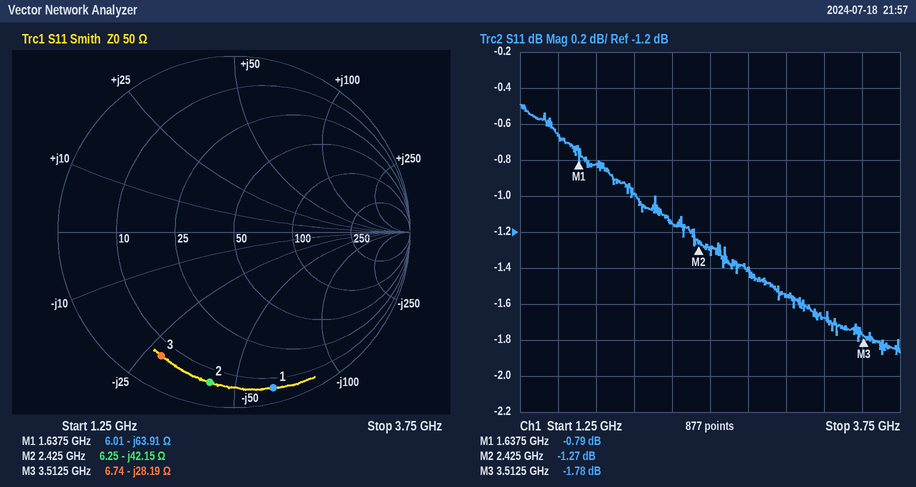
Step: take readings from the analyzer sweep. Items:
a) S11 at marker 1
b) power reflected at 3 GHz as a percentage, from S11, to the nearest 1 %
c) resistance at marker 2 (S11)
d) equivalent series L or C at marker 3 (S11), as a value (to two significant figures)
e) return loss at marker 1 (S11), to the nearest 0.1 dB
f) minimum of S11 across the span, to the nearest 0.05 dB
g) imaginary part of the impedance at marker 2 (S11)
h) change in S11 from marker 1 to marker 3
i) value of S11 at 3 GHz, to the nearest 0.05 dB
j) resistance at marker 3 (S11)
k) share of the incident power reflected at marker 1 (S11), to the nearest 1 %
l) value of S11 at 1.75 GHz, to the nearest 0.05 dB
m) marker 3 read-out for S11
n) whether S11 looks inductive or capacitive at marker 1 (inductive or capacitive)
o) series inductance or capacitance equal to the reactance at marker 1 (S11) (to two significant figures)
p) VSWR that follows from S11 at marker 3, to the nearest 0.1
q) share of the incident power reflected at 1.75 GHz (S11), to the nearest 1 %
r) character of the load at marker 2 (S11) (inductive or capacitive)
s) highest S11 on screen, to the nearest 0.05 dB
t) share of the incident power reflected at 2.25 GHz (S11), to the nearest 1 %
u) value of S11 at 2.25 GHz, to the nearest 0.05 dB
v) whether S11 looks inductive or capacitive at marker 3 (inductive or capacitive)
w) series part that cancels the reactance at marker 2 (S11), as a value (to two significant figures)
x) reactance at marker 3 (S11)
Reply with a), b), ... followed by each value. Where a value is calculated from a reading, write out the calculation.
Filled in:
a) -0.79 dB
b) 10^(-1.55/10) ≈ 70 %
c) 6.25 Ω
d) C = 1/(2π × 3.5125 GHz × 28.19 Ω) ≈ 1.6 pF
e) 0.8 dB
f) -1.90 dB
g) -42.15 Ω
h) -1.78 − (-0.79) = -0.99 dB
i) -1.55 dB
j) 6.74 Ω
k) 10^(-0.79/10) ≈ 83 %
l) -0.80 dB
m) -1.78 dB
n) capacitive
o) C = 1/(2π × 1.6375 GHz × 63.91 Ω) ≈ 1.5 pF
p) (1 + 0.8147)/(1 − 0.8147) ≈ 9.8
q) 10^(-0.8/10) ≈ 83 %
r) capacitive
s) -0.50 dB
t) 10^(-1.15/10) ≈ 77 %
u) -1.15 dB
v) capacitive
w) L = 42.15 Ω/(2π × 2.425 GHz) ≈ 2.8 nH
x) -28.19 Ω
